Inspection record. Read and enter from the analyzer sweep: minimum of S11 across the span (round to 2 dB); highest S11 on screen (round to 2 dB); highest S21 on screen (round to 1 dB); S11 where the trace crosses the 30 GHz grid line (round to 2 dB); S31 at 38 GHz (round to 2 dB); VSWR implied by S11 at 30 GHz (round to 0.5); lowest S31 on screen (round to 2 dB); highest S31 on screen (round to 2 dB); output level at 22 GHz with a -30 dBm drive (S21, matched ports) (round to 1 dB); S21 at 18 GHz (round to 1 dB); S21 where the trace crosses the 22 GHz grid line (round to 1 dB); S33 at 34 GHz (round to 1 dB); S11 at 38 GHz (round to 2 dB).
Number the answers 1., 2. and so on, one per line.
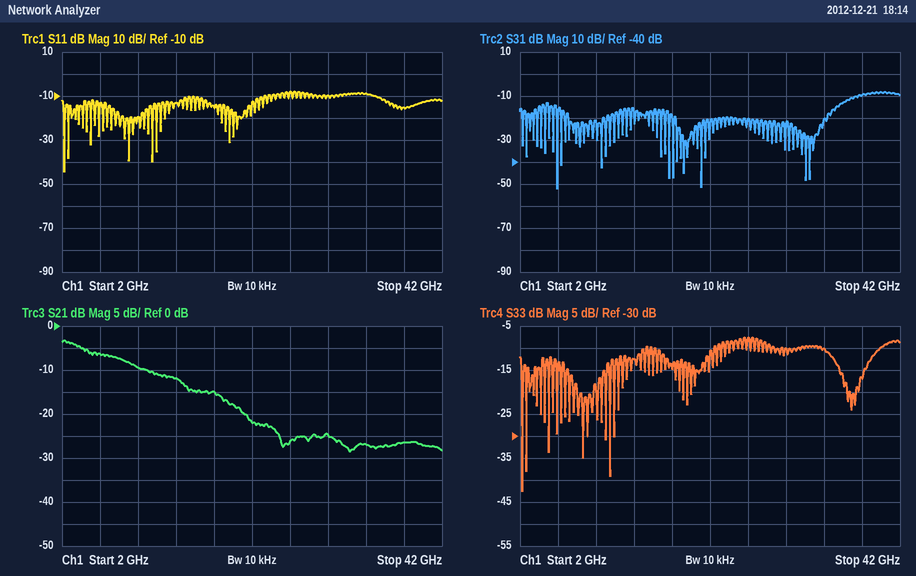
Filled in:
1. -44 dB
2. -8 dB
3. -3 dB
4. -10 dB
5. -10 dB
6. 2.0
7. -52 dB
8. -8 dB
9. -52 dBm
10. -15 dB
11. -22 dB
12. -10 dB
13. -16 dB
